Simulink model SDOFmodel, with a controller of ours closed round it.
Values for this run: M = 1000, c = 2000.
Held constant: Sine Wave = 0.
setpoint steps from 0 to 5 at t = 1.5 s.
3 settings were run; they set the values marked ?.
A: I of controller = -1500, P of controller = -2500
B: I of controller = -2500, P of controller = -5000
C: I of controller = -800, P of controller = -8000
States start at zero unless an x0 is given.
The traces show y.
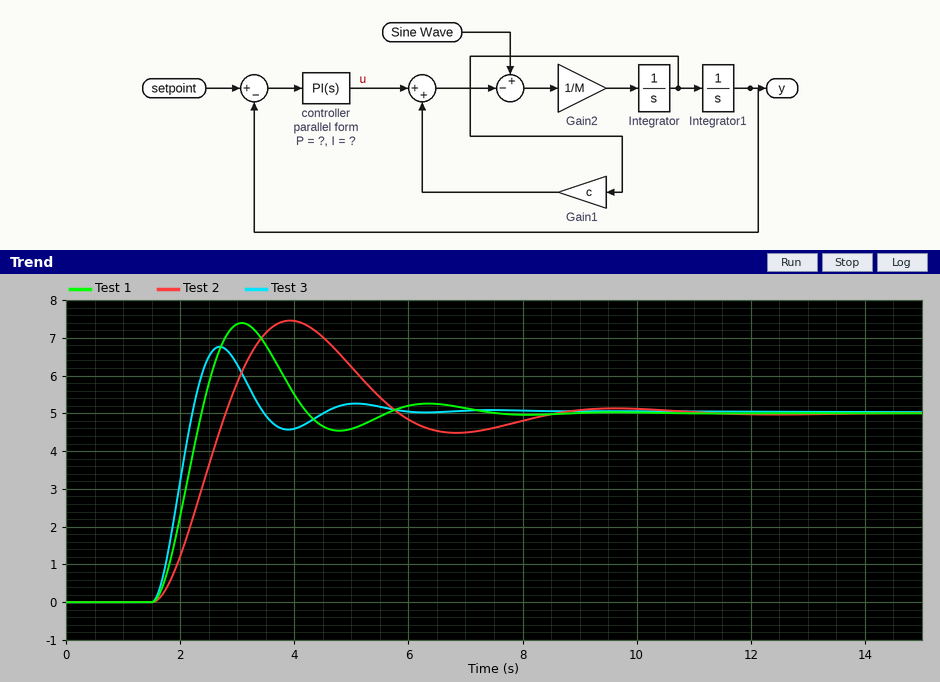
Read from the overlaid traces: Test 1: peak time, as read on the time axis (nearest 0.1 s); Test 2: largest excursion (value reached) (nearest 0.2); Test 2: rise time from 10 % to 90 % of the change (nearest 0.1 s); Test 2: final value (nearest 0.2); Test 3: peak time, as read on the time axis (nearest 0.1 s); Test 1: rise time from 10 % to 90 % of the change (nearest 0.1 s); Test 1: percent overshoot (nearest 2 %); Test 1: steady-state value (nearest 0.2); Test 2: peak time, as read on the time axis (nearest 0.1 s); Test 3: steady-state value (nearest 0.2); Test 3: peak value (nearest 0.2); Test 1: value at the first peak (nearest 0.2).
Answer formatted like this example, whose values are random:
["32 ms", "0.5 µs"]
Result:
["3.1 s", "7.4", "0.9 s", "5.0", "2.7 s", "0.6 s", "48 %", "5.0", "3.9 s", "5.0", "6.8", "7.4"]
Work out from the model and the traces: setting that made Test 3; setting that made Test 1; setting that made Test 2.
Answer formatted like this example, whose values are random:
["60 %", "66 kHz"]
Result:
["C", "B", "A"]
